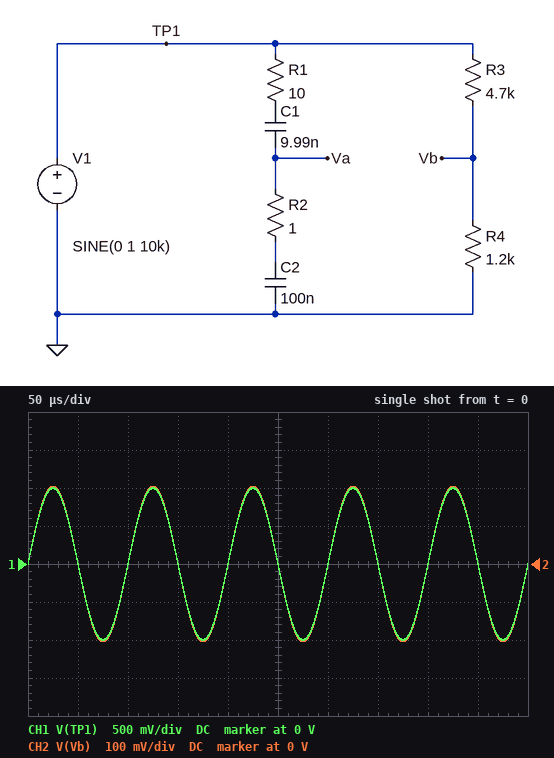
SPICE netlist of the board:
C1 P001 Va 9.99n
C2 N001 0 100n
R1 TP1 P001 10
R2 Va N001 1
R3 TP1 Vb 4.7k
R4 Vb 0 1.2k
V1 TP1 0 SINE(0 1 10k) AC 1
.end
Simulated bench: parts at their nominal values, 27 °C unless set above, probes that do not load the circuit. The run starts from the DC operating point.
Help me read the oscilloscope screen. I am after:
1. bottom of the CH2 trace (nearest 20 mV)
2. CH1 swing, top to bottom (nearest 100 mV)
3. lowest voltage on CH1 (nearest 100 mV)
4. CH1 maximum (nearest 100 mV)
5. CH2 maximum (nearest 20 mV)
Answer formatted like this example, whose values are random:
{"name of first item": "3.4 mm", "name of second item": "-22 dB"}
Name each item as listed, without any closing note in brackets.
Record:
{"bottom of the CH2 trace": "-200 mV", "CH1 swing, top to bottom": "2.0 V", "lowest voltage on CH1": "-1.0 V", "CH1 maximum": "1.0 V", "CH2 maximum": "200 mV"}
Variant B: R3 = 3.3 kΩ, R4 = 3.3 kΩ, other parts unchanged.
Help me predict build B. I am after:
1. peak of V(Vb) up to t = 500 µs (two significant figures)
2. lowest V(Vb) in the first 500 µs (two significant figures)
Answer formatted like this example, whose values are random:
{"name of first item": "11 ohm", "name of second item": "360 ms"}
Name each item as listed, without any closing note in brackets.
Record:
{"peak of V(Vb) up to t = 500 µs": "500 mV", "lowest V(Vb) in the first 500 µs": "-500 mV"}
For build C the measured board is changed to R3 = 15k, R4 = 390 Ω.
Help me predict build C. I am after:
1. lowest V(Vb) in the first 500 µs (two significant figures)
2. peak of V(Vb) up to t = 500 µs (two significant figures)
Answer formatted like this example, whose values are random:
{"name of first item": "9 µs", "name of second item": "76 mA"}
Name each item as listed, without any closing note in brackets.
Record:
{"lowest V(Vb) in the first 500 µs": "-25 mV", "peak of V(Vb) up to t = 500 µs": "25 mV"}
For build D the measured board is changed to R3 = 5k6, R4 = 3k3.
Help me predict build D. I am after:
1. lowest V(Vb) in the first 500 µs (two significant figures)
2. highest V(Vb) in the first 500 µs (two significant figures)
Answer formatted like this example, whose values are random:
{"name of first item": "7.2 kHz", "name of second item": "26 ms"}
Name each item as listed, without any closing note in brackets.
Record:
{"lowest V(Vb) in the first 500 µs": "-370 mV", "highest V(Vb) in the first 500 µs": "370 mV"}
